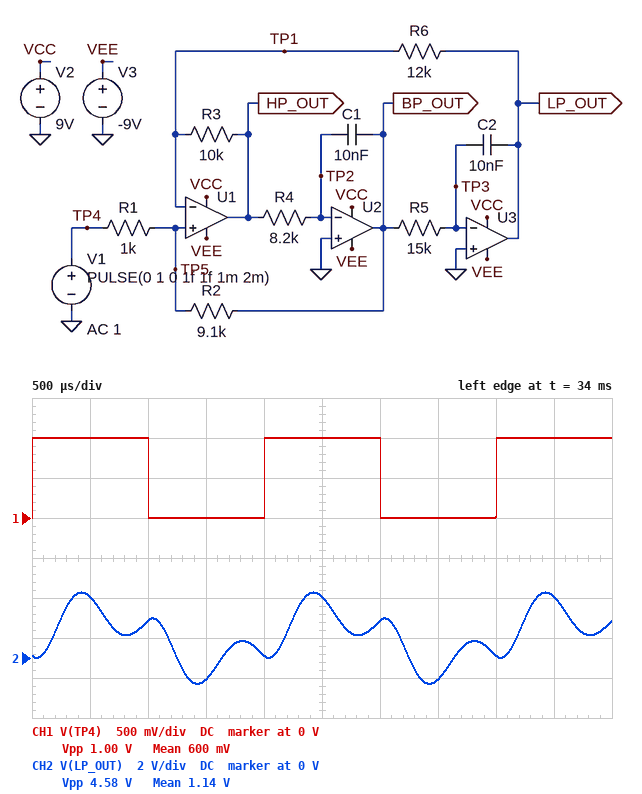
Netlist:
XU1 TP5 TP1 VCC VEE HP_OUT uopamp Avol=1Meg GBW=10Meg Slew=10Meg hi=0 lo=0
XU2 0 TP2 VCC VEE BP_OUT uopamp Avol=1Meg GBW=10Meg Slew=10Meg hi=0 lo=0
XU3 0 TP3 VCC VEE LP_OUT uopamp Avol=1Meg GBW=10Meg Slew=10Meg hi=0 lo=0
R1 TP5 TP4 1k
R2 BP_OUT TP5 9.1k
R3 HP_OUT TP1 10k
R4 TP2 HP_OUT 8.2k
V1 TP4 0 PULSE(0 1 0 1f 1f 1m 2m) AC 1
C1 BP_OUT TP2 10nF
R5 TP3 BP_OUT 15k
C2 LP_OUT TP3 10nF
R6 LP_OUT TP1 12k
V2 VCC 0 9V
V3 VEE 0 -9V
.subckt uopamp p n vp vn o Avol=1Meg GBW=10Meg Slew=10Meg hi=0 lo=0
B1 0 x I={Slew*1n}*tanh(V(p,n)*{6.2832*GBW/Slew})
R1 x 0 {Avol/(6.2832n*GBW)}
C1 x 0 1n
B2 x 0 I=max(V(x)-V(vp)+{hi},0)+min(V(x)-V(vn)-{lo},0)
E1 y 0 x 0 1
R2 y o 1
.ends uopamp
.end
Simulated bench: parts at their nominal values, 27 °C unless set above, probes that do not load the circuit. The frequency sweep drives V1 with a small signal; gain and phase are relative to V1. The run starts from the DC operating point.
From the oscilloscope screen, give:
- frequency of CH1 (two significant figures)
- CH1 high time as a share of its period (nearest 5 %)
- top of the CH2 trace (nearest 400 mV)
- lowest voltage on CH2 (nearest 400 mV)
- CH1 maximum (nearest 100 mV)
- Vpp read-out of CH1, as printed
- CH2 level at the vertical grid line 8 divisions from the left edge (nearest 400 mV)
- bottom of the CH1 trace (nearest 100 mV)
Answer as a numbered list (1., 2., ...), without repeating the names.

1. 500 Hz
2. 50 %
3. 3.2 V
4. -1.2 V
5. 1.0 V
6. 1.00 V
7. 0 V
8. 0 V
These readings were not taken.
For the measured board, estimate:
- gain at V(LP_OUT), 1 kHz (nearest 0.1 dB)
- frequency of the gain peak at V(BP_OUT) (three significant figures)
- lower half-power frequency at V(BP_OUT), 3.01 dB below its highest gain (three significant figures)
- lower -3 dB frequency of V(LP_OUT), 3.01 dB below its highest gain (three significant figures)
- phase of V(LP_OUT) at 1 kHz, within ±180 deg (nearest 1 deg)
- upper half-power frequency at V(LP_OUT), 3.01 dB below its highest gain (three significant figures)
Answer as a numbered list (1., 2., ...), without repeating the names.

1. 12.6 dB
2. 1.31 kHz
3. 1.15 kHz
4. 1.09 kHz
5. -26 deg
6. 1.45 kHz
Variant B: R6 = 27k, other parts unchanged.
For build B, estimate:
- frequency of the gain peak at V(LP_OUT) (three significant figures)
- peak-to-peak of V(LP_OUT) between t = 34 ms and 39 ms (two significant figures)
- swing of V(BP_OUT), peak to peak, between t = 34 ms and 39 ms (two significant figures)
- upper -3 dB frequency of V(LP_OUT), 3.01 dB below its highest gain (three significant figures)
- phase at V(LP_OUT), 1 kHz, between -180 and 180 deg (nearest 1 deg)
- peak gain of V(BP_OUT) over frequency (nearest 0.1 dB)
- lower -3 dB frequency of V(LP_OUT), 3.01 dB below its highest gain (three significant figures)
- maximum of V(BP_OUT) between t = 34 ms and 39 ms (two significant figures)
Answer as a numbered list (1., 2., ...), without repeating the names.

1. 853 Hz
2. 6.6 V
3. 3.5 V
4. 977 Hz
5. -132 deg
6. 19.2 dB
7. 708 Hz
8. 1.7 V
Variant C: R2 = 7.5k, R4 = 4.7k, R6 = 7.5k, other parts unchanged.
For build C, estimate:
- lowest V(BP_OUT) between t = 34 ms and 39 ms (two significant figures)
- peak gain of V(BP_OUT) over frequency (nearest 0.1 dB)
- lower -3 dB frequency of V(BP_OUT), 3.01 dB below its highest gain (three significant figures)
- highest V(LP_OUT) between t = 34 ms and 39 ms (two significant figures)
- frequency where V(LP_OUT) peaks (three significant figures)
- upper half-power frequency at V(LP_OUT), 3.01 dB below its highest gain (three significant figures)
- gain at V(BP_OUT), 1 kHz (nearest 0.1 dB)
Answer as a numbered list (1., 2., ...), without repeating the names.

1. -2.3 V
2. 17.5 dB
3. 1.77 kHz
4. 2.3 V
5. 2.09 kHz
6. 2.52 kHz
7. 5.0 dB
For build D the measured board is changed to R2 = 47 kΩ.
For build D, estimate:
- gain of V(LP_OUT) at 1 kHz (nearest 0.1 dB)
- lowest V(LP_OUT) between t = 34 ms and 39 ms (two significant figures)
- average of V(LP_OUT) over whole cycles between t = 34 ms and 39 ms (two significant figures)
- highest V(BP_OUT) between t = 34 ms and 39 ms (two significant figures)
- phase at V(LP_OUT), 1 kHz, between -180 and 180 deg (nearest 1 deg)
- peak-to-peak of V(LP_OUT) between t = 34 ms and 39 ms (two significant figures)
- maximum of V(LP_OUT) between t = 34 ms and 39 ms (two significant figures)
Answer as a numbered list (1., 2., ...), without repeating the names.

1. 14.2 dB
2. -1.9 V
3. 1.1 V
4. 2.4 V
5. -6 deg
6. 5.9 V
7. 4.0 V
